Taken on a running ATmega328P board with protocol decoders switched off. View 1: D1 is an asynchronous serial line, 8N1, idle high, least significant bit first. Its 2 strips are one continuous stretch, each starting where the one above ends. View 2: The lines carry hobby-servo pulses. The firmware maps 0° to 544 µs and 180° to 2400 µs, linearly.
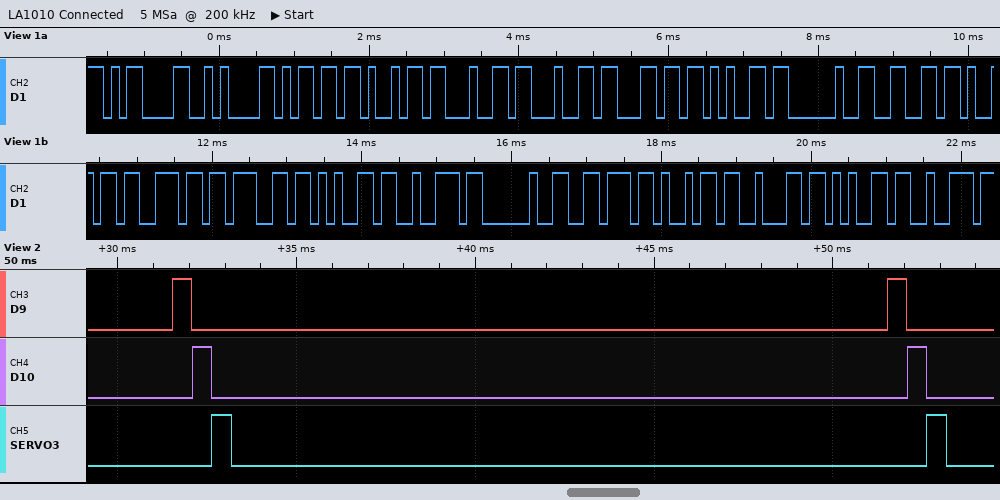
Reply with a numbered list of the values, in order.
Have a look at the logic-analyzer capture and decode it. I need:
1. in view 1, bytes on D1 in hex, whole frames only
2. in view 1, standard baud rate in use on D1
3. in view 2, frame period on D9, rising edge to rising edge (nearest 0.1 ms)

1. 0x0D 0x0A 0x6D 0x69 0x64 0x64 0x6C 0x65 0x20 0x66 0x69 0x6E 0x67 0x65 0x72 0x20 0x76 0x69 0x62 0x65 0x72
2. 9600 baud
3. 20.0 ms
